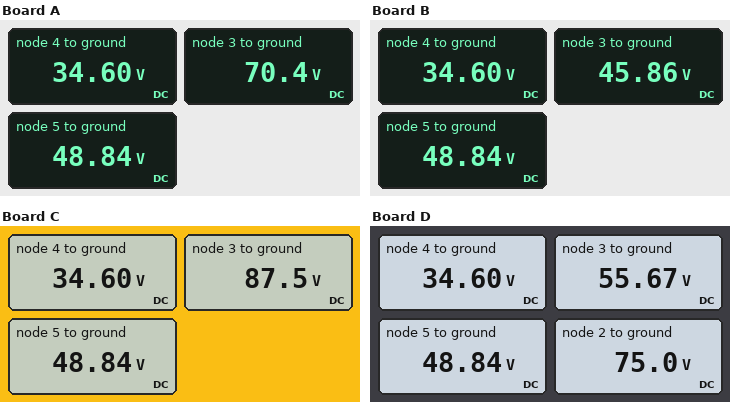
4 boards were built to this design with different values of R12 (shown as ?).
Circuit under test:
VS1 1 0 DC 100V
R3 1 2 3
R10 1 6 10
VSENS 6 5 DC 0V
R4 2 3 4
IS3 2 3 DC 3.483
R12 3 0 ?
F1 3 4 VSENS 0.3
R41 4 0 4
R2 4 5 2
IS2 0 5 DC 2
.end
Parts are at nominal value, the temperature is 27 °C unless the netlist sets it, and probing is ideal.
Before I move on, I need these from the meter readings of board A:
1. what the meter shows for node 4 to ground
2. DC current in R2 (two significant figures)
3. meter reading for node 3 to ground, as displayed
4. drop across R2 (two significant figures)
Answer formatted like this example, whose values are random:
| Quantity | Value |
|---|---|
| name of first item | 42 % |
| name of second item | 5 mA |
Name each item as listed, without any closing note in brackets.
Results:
| Quantity | Value |
|---|---|
| what the meter shows for node 4 to ground | 34.60 V |
| DC current in R2 | 7.1 A |
| meter reading for node 3 to ground, as displayed | 70.4 V |
| drop across R2 | 14 V |
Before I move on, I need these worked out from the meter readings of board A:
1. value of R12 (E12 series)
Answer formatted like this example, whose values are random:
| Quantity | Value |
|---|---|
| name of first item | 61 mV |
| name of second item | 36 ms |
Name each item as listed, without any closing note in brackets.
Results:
| Quantity | Value |
|---|---|
| value of R12 | 15 Ω |
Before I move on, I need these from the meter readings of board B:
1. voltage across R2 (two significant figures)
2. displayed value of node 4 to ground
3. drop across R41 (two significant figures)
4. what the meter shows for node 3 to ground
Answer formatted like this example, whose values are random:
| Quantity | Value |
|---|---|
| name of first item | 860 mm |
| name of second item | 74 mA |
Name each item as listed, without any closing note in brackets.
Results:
| Quantity | Value |
|---|---|
| voltage across R2 | 14 V |
| displayed value of node 4 to ground | 34.60 V |
| drop across R41 | 35 V |
| what the meter shows for node 3 to ground | 45.86 V |
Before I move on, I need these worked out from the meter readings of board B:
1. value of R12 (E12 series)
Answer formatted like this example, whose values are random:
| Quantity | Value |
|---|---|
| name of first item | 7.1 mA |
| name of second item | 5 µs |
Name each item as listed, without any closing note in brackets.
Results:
| Quantity | Value |
|---|---|
| value of R12 | 5.6 Ω |
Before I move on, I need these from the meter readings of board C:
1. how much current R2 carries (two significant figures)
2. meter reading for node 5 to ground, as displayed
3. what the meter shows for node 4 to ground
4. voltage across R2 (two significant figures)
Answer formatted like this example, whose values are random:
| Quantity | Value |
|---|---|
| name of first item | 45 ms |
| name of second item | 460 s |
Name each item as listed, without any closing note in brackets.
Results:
| Quantity | Value |
|---|---|
| how much current R2 carries | 7.1 A |
| meter reading for node 5 to ground, as displayed | 48.84 V |
| what the meter shows for node 4 to ground | 34.60 V |
| voltage across R2 | 14 V |
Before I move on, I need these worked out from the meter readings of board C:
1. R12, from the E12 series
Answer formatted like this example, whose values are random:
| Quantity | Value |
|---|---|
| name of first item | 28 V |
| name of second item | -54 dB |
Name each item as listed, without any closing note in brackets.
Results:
| Quantity | Value |
|---|---|
| R12, from the E12 series | 39 Ω |
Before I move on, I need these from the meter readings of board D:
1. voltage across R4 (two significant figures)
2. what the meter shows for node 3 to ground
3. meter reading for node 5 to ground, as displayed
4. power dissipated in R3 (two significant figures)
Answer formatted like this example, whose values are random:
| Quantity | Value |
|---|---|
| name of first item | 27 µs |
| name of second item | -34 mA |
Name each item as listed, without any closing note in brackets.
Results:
| Quantity | Value |
|---|---|
| voltage across R4 | 19 V |
| what the meter shows for node 3 to ground | 55.67 V |
| meter reading for node 5 to ground, as displayed | 48.84 V |
| power dissipated in R3 | 210 W |
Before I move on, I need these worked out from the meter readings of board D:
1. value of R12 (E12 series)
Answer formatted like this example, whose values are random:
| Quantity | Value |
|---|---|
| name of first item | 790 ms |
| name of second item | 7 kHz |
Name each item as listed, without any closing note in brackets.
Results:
| Quantity | Value |
|---|---|
| value of R12 | 8.2 Ω |
